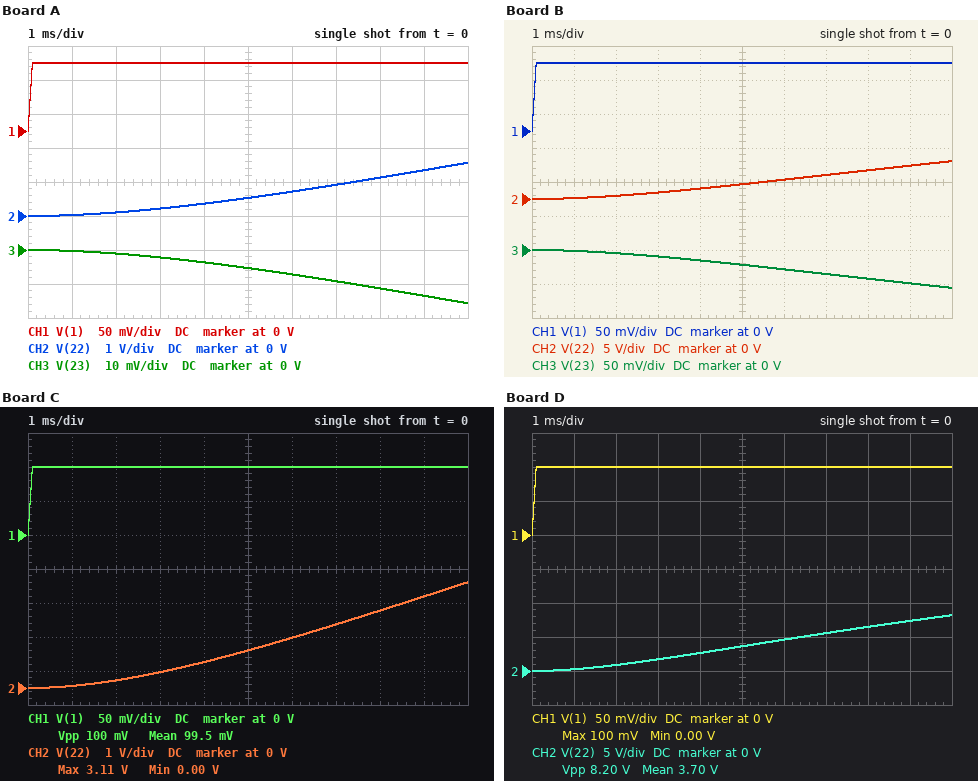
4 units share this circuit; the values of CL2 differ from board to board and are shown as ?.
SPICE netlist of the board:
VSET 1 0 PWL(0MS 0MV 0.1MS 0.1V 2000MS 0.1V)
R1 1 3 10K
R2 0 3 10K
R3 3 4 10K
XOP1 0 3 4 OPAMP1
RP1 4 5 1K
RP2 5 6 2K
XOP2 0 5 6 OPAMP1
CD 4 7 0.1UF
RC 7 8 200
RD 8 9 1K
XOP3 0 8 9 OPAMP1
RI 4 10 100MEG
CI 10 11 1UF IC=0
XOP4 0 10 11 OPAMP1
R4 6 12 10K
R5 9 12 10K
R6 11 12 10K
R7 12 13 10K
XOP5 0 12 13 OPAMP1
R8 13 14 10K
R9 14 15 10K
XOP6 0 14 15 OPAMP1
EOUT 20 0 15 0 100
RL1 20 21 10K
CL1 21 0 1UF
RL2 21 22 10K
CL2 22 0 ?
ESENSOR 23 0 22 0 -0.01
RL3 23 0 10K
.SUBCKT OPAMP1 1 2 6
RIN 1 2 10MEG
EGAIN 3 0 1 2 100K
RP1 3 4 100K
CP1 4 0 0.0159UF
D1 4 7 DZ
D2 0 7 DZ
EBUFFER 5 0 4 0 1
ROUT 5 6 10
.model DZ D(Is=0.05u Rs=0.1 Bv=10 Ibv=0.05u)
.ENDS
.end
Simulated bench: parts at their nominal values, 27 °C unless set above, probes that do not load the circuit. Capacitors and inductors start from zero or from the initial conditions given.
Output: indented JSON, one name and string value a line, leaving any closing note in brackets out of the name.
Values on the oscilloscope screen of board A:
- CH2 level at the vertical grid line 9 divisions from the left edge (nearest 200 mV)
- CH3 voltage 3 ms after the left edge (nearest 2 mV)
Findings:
{
  "CH2 level at the vertical grid line 9 divisions from the left edge": "1.4 V",
  "CH3 voltage 3 ms after the left edge": "-2 mV"
}
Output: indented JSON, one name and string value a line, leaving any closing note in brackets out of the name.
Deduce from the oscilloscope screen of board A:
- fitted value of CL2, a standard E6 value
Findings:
{
  "fitted value of CL2, a standard E6 value": "3.3 µF"
}
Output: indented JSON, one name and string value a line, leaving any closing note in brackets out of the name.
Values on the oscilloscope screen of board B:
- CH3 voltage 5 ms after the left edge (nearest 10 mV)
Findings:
{
  "CH3 voltage 5 ms after the left edge": "-20 mV"
}
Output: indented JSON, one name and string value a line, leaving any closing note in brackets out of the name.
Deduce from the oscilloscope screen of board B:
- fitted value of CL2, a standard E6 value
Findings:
{
  "fitted value of CL2, a standard E6 value": "680 nF"
}
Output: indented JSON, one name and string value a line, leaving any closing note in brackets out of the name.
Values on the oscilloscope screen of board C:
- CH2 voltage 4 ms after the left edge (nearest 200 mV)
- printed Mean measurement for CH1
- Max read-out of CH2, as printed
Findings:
{
  "CH2 voltage 4 ms after the left edge": "800 mV",
  "printed Mean measurement for CH1": "99.5 mV",
  "Max read-out of CH2, as printed": "3.11 V"
}
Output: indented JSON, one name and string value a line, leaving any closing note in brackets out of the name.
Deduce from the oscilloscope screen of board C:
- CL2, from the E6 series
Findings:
{
  "CL2, from the E6 series": "1.5 µF"
}
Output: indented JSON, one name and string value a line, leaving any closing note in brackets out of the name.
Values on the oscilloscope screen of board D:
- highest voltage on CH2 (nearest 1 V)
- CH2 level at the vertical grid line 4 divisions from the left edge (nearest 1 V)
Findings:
{
  "highest voltage on CH2": "8 V",
  "CH2 level at the vertical grid line 4 divisions from the left edge": "3 V"
}
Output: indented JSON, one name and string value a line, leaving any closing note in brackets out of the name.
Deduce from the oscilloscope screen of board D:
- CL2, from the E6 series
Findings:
{
  "CL2, from the E6 series": "330 nF"
}
